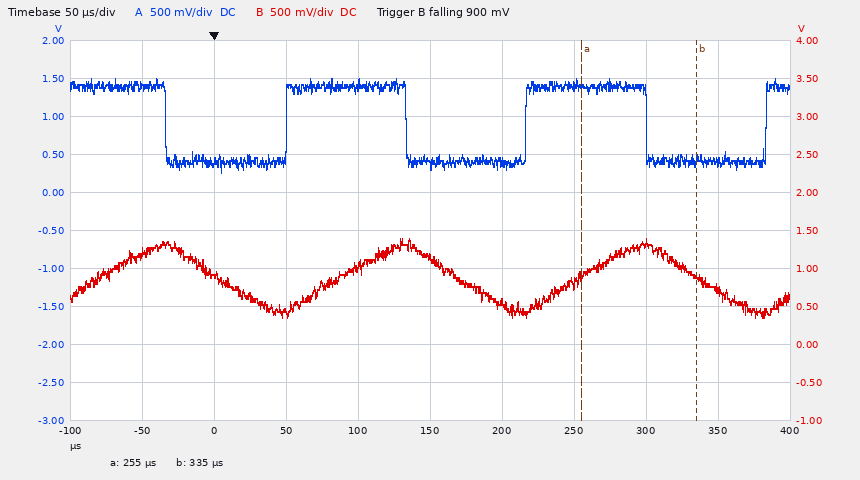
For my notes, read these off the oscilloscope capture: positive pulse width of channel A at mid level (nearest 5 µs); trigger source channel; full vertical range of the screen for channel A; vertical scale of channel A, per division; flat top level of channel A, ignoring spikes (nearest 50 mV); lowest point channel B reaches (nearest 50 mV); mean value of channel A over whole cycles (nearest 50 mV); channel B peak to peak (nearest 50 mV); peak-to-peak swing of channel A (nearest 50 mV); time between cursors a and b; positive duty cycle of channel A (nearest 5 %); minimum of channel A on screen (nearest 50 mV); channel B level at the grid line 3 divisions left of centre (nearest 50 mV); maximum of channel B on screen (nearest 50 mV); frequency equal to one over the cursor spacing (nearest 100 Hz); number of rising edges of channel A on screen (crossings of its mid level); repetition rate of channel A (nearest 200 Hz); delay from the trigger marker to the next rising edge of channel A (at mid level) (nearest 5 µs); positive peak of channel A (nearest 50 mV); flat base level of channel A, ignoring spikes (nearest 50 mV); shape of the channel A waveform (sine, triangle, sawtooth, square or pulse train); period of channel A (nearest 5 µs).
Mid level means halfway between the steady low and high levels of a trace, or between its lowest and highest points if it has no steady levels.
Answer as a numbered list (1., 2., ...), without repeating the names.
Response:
1. 85 µs
2. channel B
3. 5 V
4. 500 mV
5. 1.40 V
6. 350 mV
7. 900 mV
8. 1.05 V
9. 1.25 V
10. 80 µs
11. 50 %
12. 250 mV
13. 900 mV
14. 1.40 V
15. 12.5 kHz
16. 3
17. 6.0 kHz
18. 50 µs
19. 1.50 V
20. 400 mV
21. square
22. 165 µs
